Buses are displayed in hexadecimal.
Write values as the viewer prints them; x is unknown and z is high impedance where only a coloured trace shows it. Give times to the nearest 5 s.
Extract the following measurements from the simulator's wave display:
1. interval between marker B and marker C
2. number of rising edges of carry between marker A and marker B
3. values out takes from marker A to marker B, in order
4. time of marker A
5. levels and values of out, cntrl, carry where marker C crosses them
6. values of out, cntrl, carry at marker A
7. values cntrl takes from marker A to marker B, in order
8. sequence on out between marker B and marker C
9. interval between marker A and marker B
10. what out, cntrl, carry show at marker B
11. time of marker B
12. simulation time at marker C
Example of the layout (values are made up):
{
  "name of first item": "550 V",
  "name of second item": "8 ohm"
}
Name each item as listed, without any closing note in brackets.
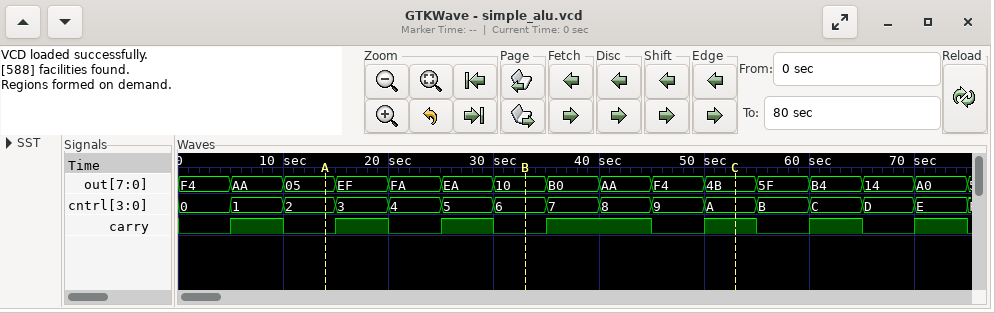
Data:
{
  "interval between marker B and marker C": "20 s",
  "number of rising edges of carry between marker A and marker B": "2",
  "values out takes from marker A to marker B, in order": "05, EF, FA, EA, 10",
  "time of marker A": "15 s",
  "levels and values of out, cntrl, carry where marker C crosses them": "out=4B, cntrl=A, carry=1",
  "values of out, cntrl, carry at marker A": "out=05, cntrl=2, carry=0",
  "values cntrl takes from marker A to marker B, in order": "2, 3, 4, 5, 6",
  "sequence on out between marker B and marker C": "10, B0, AA, F4, 4B",
  "interval between marker A and marker B": "20 s",
  "what out, cntrl, carry show at marker B": "out=10, cntrl=6, carry=0",
  "time of marker B": "35 s",
  "simulation time at marker C": "55 s"
}
